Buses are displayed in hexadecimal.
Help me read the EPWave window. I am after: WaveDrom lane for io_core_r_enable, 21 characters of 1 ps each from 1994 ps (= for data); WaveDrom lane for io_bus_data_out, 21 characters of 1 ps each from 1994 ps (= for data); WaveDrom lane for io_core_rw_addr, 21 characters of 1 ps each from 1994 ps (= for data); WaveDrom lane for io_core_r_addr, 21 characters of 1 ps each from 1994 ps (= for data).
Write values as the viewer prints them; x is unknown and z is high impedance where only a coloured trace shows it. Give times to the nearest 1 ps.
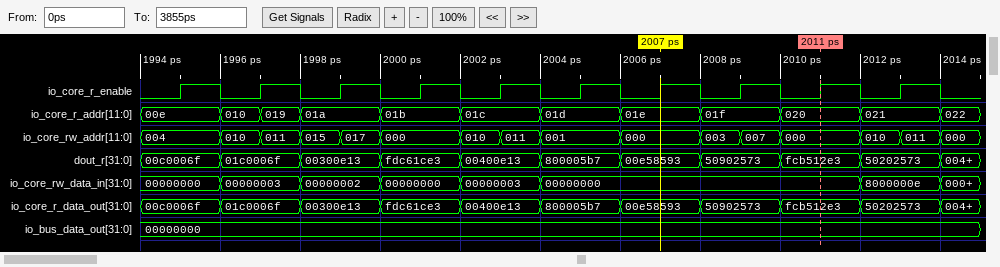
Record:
{name: 'io_core_r_enable', wave: '010101010101010101010'}
{name: 'io_bus_data_out', wave: '=....................', data: '00000000'}
{name: 'io_core_rw_addr', wave: '=.=====.===.=.===.===', data: '004 010 011 015 017 000 010 011 001 000 003 007 000 010 011 000'}
{name: 'io_core_r_addr', wave: '=.===.=.=.=.=.=.=.=.=', data: '00e 010 019 01a 01b 01c 01d 01e 01f 020 021 022'}
